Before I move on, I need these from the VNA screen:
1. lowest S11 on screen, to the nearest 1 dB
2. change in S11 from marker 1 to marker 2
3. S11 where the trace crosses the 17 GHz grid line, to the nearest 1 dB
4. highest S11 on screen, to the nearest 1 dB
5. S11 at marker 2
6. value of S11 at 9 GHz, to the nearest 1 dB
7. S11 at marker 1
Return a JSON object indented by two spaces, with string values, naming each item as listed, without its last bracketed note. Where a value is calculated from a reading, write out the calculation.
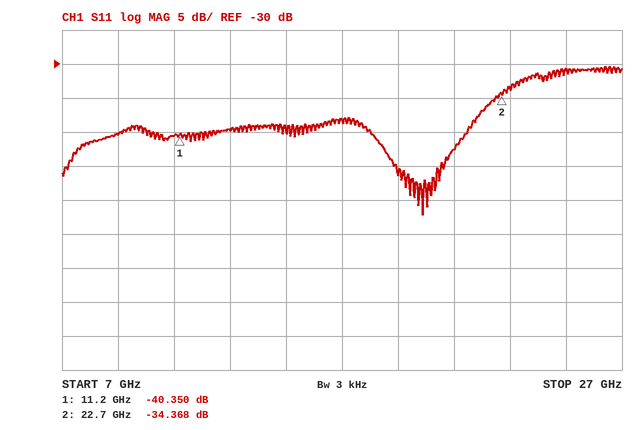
{
  "lowest S11 on screen, to the nearest 1 dB": "-52 dB",
  "change in S11 from marker 1 to marker 2": "-34.368 − (-40.35) = 5.982 dB",
  "S11 where the trace crosses the 17 GHz grid line, to the nearest 1 dB": "-38 dB",
  "highest S11 on screen, to the nearest 1 dB": "-30 dB",
  "S11 at marker 2": "-34.368 dB",
  "value of S11 at 9 GHz, to the nearest 1 dB": "-40 dB",
  "S11 at marker 1": "-40.350 dB"
}
